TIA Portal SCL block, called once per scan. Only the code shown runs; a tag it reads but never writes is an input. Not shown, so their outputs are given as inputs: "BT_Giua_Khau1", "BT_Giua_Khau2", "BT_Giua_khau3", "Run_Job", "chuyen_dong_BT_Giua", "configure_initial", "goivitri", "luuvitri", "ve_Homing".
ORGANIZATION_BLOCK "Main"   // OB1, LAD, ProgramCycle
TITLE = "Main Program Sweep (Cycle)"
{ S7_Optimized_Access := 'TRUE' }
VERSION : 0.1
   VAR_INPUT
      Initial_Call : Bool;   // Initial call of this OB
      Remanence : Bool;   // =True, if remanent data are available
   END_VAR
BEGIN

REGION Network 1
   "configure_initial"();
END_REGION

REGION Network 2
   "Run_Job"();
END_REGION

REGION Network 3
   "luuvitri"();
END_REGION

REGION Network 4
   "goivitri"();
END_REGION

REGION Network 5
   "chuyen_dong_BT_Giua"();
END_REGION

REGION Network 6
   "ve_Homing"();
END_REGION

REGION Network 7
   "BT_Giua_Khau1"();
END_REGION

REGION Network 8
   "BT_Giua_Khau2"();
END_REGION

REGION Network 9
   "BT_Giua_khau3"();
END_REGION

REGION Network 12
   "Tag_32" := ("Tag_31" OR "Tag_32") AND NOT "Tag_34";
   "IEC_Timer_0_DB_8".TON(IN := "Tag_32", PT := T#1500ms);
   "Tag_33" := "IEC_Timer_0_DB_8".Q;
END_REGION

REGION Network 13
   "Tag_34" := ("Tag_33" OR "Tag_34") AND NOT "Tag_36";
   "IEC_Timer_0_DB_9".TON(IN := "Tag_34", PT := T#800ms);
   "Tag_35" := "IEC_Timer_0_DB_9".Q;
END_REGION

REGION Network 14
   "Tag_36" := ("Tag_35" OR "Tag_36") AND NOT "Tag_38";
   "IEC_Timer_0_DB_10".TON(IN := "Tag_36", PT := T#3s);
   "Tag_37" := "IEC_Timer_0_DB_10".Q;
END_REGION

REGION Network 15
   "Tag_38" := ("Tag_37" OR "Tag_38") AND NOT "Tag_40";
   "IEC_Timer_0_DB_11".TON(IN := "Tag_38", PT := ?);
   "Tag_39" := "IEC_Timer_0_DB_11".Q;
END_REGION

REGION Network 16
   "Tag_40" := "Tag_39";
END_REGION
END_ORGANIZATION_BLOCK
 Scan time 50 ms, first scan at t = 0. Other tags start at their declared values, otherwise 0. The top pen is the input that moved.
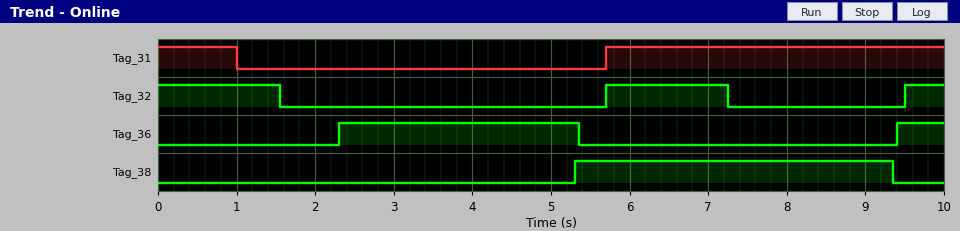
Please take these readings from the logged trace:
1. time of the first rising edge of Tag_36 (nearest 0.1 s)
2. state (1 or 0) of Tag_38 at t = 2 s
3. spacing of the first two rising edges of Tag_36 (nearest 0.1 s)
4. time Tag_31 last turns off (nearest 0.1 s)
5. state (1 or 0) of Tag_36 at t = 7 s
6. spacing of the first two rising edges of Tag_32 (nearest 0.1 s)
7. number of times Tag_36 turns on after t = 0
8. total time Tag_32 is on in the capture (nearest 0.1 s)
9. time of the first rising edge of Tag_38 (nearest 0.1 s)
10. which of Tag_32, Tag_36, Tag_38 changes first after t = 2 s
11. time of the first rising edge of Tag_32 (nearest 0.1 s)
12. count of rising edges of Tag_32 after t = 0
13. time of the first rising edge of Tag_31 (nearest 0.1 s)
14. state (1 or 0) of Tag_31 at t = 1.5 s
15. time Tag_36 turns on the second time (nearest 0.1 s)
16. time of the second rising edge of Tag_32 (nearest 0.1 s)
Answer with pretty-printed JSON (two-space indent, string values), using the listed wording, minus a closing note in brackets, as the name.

{
  "time of the first rising edge of Tag_36": "2.3 s",
  "state (1 or 0) of Tag_38 at t = 2 s": "0",
  "spacing of the first two rising edges of Tag_36": "7.1 s",
  "time Tag_31 last turns off": "1.0 s",
  "state (1 or 0) of Tag_36 at t = 7 s": "0",
  "spacing of the first two rising edges of Tag_32": "3.8 s",
  "number of times Tag_36 turns on after t = 0": "2",
  "total time Tag_32 is on in the capture": "3.6 s",
  "time of the first rising edge of Tag_38": "5.3 s",
  "which of Tag_32, Tag_36, Tag_38 changes first after t = 2 s": "Tag_36",
  "time of the first rising edge of Tag_32": "5.7 s",
  "count of rising edges of Tag_32 after t = 0": "2",
  "time of the first rising edge of Tag_31": "5.7 s",
  "state (1 or 0) of Tag_31 at t = 1.5 s": "0",
  "time Tag_36 turns on the second time": "9.4 s",
  "time of the second rising edge of Tag_32": "9.5 s"
}
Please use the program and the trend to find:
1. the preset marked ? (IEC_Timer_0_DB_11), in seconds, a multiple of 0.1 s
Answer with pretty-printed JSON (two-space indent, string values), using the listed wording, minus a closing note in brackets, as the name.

{
  "the preset marked ? (IEC_Timer_0_DB_11), in seconds, a multiple of 0.1 s": "4.0 s"
}
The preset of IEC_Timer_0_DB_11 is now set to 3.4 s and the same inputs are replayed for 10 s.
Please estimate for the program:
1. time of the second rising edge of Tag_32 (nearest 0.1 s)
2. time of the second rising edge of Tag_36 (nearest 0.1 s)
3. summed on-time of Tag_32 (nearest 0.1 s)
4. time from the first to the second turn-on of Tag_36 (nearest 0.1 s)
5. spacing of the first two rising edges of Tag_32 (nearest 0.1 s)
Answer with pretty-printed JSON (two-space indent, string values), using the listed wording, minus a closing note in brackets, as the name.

{
  "time of the second rising edge of Tag_32": "8.9 s",
  "time of the second rising edge of Tag_36": "8.8 s",
  "summed on-time of Tag_32": "4.2 s",
  "time from the first to the second turn-on of Tag_36": "6.5 s",
  "spacing of the first two rising edges of Tag_32": "3.2 s"
}
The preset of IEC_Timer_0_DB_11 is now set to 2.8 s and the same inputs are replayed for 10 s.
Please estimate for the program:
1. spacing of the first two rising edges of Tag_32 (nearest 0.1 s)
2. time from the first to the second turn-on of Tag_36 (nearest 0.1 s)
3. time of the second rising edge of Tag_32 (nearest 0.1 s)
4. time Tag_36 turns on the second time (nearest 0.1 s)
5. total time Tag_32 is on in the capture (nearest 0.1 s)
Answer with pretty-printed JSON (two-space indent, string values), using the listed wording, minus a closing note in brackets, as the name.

{
  "spacing of the first two rising edges of Tag_32": "2.6 s",
  "time from the first to the second turn-on of Tag_36": "5.9 s",
  "time of the second rising edge of Tag_32": "8.3 s",
  "time Tag_36 turns on the second time": "8.2 s",
  "total time Tag_32 is on in the capture": "4.8 s"
}
